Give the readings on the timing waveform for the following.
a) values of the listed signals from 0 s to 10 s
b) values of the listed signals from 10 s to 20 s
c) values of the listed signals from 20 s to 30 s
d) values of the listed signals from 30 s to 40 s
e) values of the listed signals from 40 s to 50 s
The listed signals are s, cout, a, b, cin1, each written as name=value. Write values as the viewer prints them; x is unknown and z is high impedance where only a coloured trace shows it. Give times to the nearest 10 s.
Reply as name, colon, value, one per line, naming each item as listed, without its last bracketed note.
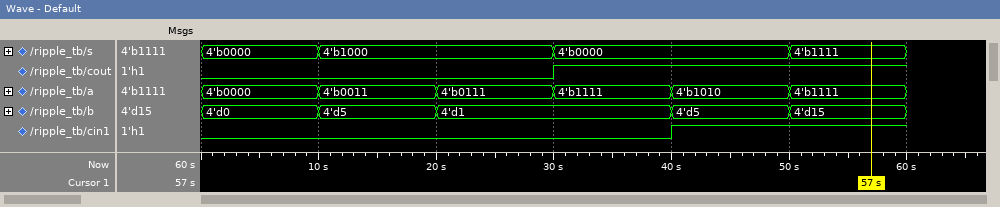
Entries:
values of the listed signals from 0 s to 10 s: s=4'b0000, cout=0, a=4'b0000, b=4'd0, cin1=0
values of the listed signals from 10 s to 20 s: s=4'b1000, cout=0, a=4'b0011, b=4'd5, cin1=0
values of the listed signals from 20 s to 30 s: s=4'b1000, cout=0, a=4'b0111, b=4'd1, cin1=0
values of the listed signals from 30 s to 40 s: s=4'b0000, cout=1, a=4'b1111, b=4'd1, cin1=0
values of the listed signals from 40 s to 50 s: s=4'b0000, cout=1, a=4'b1010, b=4'd5, cin1=1
